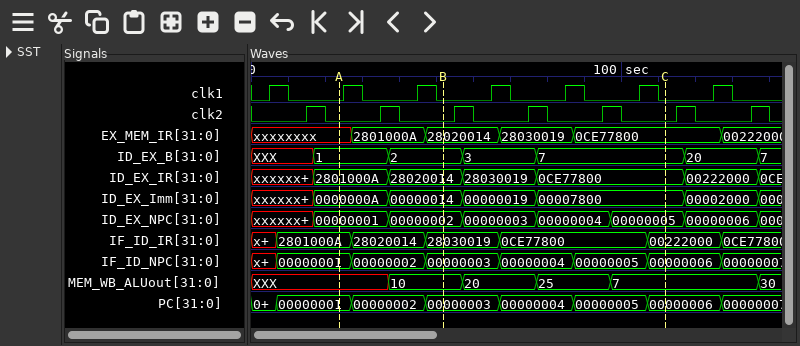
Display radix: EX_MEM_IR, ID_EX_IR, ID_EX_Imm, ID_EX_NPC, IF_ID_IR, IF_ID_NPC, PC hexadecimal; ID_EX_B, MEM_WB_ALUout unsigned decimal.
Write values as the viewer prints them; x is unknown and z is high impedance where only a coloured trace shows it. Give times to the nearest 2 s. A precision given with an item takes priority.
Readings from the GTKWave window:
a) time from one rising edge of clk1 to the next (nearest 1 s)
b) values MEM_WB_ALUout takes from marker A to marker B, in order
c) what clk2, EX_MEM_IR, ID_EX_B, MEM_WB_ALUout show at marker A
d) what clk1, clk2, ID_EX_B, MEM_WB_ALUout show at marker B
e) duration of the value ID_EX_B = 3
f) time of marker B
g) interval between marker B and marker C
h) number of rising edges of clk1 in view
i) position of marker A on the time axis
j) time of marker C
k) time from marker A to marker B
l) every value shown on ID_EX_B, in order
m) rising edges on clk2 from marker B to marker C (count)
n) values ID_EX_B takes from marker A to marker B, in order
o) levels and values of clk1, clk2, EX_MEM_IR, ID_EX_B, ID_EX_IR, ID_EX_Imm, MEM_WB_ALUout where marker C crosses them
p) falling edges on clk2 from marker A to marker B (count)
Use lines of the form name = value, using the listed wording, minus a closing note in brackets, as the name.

time from one rising edge of clk1 to the next = 20 s
values MEM_WB_ALUout takes from marker A to marker B, in order = XXX, 10
what clk2, EX_MEM_IR, ID_EX_B, MEM_WB_ALUout show at marker A = clk2=0, EX_MEM_IR=xxxxxxxx, ID_EX_B=1, MEM_WB_ALUout=XXX
what clk1, clk2, ID_EX_B, MEM_WB_ALUout show at marker B = clk1=0, clk2=0, ID_EX_B=2, MEM_WB_ALUout=10
duration of the value ID_EX_B = 3 = 20 s
time of marker B = 52 s
interval between marker B and marker C = 60 s
number of rising edges of clk1 in view = 7
position of marker A on the time axis = 24 s
time of marker C = 112 s
time from marker A to marker B = 28 s
every value shown on ID_EX_B, in order = XXX, 1, 2, 3, 7, 20, 7
rising edges on clk2 from marker B to marker C = 3
values ID_EX_B takes from marker A to marker B, in order = 1, 2
levels and values of clk1, clk2, EX_MEM_IR, ID_EX_B, ID_EX_IR, ID_EX_Imm, MEM_WB_ALUout where marker C crosses them = clk1=0, clk2=0, EX_MEM_IR=0CE77800, ID_EX_B=7, ID_EX_IR=0CE77800, ID_EX_Imm=00007800, MEM_WB_ALUout=7
falling edges on clk2 from marker A to marker B = 1
